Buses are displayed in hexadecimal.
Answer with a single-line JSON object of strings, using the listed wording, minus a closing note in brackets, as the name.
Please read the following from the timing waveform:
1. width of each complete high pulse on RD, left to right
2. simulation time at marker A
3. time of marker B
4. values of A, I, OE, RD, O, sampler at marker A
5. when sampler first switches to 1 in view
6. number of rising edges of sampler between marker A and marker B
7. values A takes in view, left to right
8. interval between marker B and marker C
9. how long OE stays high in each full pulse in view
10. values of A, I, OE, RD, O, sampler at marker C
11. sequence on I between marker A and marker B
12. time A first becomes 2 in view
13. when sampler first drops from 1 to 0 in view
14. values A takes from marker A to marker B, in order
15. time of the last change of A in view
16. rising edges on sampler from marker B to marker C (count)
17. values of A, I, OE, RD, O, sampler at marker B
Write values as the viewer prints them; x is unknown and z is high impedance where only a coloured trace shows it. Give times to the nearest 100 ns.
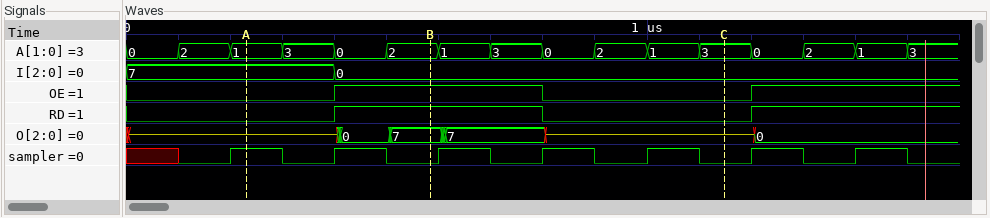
{"width of each complete high pulse on RD, left to right": "400 ns", "simulation time at marker A": "200 ns", "time of marker B": "600 ns", "values of A, I, OE, RD, O, sampler at marker A": "A=1, I=7, OE=0, RD=0, O=z, sampler=1", "when sampler first switches to 1 in view": "200 ns", "number of rising edges of sampler between marker A and marker B": "1", "values A takes in view, left to right": "0, 2, 1, 3, 0, 2, 1, 3, 0, 2, 1, 3, 0, 2, 1, 3", "interval between marker B and marker C": "600 ns", "how long OE stays high in each full pulse in view": "400 ns", "values of A, I, OE, RD, O, sampler at marker C": "A=3, I=0, OE=0, RD=0, O=z, sampler=0", "sequence on I between marker A and marker B": "7, 0", "time A first becomes 2 in view": "100 ns", "when sampler first drops from 1 to 0 in view": "300 ns", "values A takes from marker A to marker B, in order": "1, 3, 0, 2", "time of the last change of A in view": "1500 ns", "rising edges on sampler from marker B to marker C": "3", "values of A, I, OE, RD, O, sampler at marker B": "A=2, I=0, OE=1, RD=1, O=7, sampler=0"}
